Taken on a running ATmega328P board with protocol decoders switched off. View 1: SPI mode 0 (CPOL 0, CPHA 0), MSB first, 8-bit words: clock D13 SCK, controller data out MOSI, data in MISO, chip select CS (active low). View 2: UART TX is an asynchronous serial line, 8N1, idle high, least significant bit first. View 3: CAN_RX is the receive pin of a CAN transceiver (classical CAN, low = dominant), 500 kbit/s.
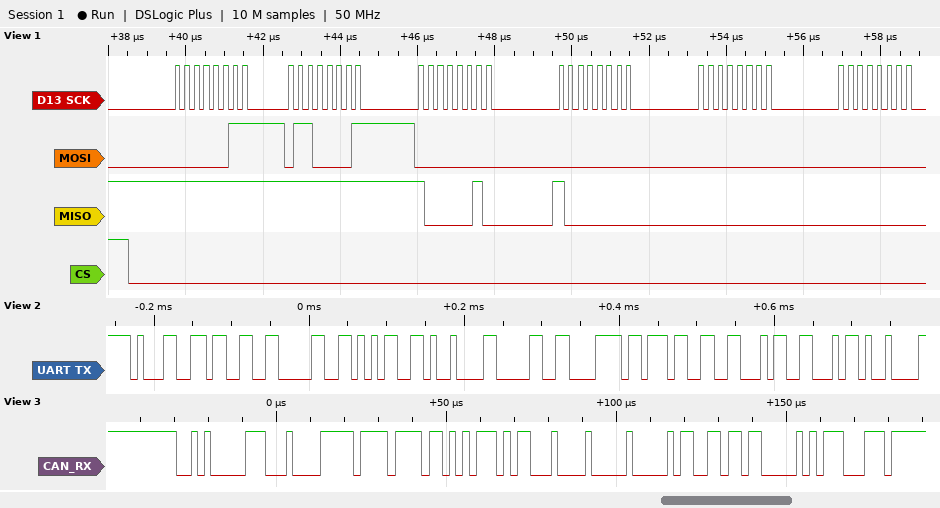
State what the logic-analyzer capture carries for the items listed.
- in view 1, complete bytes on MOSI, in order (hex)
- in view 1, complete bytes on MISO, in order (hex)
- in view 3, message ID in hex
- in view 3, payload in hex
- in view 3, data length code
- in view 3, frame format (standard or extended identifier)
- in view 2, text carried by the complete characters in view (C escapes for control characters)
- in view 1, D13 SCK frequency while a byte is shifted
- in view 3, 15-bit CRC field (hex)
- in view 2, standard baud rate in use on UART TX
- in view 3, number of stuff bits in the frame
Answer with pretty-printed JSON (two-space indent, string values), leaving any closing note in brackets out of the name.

{
  "in view 1, complete bytes on MOSI, in order": "03 61 00 00 00 00",
  "in view 1, complete bytes on MISO, in order": "FF FF 82 80 00 00",
  "in view 3, message ID in hex": "0x283",
  "in view 3, payload in hex": "7F DE D5 D6 21 00 19 B6",
  "in view 3, data length code": "8",
  "in view 3, frame format": "standard",
  "in view 2, text carried by the complete characters in view": "\"1305\\t0x7FF\\t\"",
  "in view 1, D13 SCK frequency while a byte is shifted": "4 MHz",
  "in view 3, 15-bit CRC field": "0x02E3",
  "in view 2, standard baud rate in use on UART TX": "115200 baud",
  "in view 3, number of stuff bits in the frame": "5"
}
